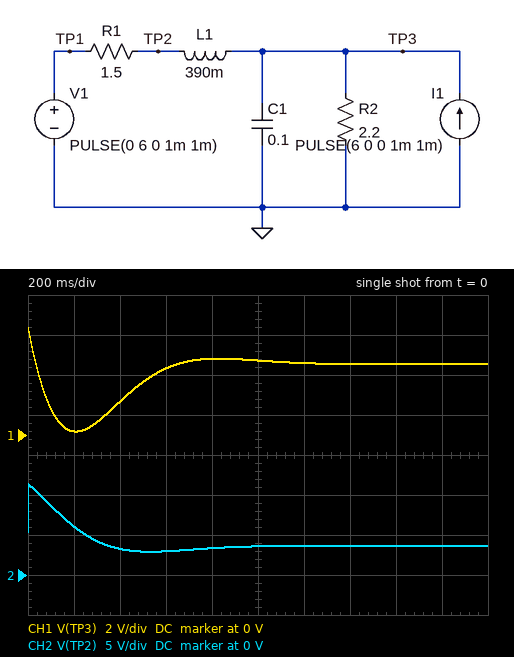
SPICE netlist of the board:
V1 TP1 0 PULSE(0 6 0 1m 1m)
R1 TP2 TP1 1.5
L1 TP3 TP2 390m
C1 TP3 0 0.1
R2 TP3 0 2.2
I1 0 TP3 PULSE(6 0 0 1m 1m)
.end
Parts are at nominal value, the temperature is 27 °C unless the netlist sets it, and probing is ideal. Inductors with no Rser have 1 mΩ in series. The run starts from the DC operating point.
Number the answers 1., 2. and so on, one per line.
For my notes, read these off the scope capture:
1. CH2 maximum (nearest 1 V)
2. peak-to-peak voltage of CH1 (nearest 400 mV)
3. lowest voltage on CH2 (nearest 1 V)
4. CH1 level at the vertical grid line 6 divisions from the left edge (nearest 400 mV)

1. 11 V
2. 5.2 V
3. 3 V
4. 3.6 V
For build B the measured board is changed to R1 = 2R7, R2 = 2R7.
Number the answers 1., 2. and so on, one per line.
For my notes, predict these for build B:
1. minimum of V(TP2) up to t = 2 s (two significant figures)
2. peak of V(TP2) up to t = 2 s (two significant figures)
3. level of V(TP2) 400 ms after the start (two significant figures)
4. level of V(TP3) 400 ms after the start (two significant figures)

1. 2.6 V
2. 14 V
3. 3.0 V
4. 2.0 V
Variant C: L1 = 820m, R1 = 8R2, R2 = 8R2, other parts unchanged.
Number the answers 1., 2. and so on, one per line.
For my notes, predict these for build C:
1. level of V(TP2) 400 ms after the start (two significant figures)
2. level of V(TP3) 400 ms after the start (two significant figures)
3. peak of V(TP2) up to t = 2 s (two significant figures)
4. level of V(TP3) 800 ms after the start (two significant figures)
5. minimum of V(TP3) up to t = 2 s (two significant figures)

1. 13 V
2. 9.8 V
3. 31 V
4. 5.1 V
5. 3.1 V
